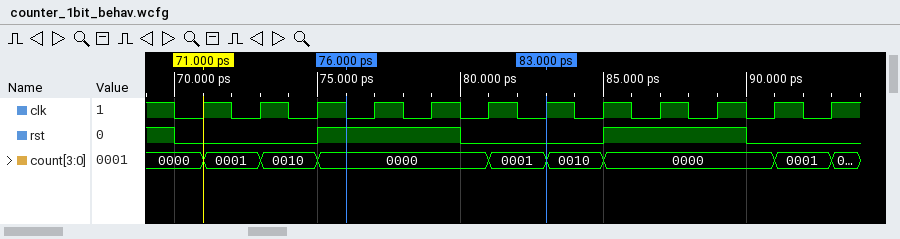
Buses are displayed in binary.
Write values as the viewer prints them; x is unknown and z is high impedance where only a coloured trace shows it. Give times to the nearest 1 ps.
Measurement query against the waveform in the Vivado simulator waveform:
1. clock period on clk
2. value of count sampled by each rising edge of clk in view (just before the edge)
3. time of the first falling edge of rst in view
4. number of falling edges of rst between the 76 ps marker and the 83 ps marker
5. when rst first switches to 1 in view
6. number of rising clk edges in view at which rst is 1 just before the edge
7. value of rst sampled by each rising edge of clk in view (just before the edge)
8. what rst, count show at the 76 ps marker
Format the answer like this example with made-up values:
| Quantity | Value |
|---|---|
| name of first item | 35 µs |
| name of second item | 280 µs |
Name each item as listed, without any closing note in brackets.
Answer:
| Quantity | Value |
|---|---|
| clock period on clk | 2 ps |
| value of count sampled by each rising edge of clk in view | 0000, 0001, 0010, 0000, 0000, 0000, 0001, 0010, 0000, 0000, 0000, 0001 |
| time of the first falling edge of rst in view | 70 ps |
| number of falling edges of rst between the 76 ps marker and the 83 ps marker | 1 |
| when rst first switches to 1 in view | 75 ps |
| number of rising clk edges in view at which rst is 1 just before the edge | 4 |
| value of rst sampled by each rising edge of clk in view | 0 0 0 1 1 0 0 0 1 1 0 0 |
| what rst, count show at the 76 ps marker | rst=1, count=0000 |
